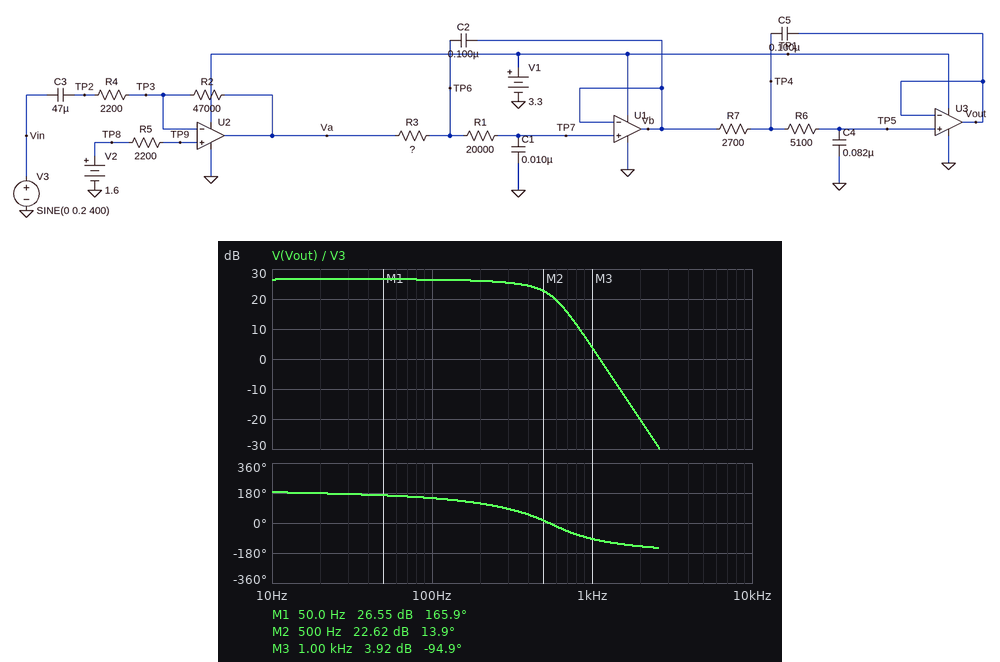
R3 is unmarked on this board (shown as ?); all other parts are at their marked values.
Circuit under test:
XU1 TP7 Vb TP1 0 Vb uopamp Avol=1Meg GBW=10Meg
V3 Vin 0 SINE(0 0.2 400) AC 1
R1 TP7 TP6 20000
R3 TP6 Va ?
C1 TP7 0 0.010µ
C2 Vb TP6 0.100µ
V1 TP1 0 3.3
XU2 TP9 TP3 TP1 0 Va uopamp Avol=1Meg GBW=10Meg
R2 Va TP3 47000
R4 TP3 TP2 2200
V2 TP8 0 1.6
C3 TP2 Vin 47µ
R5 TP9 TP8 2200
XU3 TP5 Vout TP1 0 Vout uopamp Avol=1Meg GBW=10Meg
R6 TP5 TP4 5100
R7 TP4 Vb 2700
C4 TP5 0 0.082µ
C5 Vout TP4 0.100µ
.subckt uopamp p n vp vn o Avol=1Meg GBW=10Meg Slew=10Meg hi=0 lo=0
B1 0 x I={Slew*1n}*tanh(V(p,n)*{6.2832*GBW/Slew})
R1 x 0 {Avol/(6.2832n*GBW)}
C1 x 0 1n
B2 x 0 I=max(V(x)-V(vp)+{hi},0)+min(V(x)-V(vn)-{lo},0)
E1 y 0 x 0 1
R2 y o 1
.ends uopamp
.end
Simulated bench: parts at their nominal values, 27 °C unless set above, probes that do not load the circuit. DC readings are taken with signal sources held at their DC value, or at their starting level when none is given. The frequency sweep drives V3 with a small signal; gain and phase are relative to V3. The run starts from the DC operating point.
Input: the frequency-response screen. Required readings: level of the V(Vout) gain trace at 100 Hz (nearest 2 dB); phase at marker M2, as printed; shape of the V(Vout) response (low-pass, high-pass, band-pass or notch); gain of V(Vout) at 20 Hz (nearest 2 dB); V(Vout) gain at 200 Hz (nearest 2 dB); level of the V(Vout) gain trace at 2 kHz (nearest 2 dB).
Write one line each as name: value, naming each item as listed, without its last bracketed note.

level of the V(Vout) gain trace at 100 Hz: 26 dB
phase at marker M2, as printed: 13.9 deg
shape of the V(Vout) response: low-pass
gain of V(Vout) at 20 Hz: 26 dB
V(Vout) gain at 200 Hz: 26 dB
level of the V(Vout) gain trace at 2 kHz: -20 dB
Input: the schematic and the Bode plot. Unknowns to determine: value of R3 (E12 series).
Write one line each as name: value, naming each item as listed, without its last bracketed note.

value of R3: 3.9 kΩ
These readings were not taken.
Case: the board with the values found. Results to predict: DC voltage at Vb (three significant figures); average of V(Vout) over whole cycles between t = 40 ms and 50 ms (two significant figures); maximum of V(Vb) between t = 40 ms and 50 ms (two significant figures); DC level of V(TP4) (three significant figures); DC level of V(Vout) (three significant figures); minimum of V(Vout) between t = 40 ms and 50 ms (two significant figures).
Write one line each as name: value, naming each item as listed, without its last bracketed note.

DC voltage at Vb: 1.60 V
average of V(Vout) over whole cycles between t = 40 ms and 50 ms: 1.6 V
maximum of V(Vb) between t = 40 ms and 50 ms: 3.3 V
DC level of V(TP4): 1.60 V
DC level of V(Vout): 1.60 V
minimum of V(Vout) between t = 40 ms and 50 ms: 420 mV
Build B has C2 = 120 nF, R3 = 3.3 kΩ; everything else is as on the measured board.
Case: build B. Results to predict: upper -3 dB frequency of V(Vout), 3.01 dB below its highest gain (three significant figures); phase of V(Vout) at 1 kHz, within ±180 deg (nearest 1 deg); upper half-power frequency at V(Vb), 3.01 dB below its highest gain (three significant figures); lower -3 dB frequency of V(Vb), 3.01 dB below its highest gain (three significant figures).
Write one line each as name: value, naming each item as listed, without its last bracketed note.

upper -3 dB frequency of V(Vout), 3.01 dB below its highest gain: 468 Hz
phase of V(Vout) at 1 kHz, within ±180 deg: -96 deg
upper half-power frequency at V(Vb), 3.01 dB below its highest gain: 672 Hz
lower -3 dB frequency of V(Vb), 3.01 dB below its highest gain: 4.17 Hz
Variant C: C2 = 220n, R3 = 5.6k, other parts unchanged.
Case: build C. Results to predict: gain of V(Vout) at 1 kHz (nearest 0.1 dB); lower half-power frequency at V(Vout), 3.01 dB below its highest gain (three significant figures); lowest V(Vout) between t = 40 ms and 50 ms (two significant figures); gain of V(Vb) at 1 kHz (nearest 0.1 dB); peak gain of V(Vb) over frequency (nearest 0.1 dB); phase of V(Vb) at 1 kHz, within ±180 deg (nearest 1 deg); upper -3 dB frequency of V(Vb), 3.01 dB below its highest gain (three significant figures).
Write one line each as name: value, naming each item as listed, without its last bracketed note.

gain of V(Vout) at 1 kHz: -6.9 dB
lower half-power frequency at V(Vout), 3.01 dB below its highest gain: 114 Hz
lowest V(Vout) between t = 40 ms and 50 ms: 530 mV
gain of V(Vb) at 1 kHz: 7.6 dB
peak gain of V(Vb) over frequency: 32.6 dB
phase of V(Vb) at 1 kHz, within ±180 deg: 10 deg
upper -3 dB frequency of V(Vb), 3.01 dB below its highest gain: 375 Hz
